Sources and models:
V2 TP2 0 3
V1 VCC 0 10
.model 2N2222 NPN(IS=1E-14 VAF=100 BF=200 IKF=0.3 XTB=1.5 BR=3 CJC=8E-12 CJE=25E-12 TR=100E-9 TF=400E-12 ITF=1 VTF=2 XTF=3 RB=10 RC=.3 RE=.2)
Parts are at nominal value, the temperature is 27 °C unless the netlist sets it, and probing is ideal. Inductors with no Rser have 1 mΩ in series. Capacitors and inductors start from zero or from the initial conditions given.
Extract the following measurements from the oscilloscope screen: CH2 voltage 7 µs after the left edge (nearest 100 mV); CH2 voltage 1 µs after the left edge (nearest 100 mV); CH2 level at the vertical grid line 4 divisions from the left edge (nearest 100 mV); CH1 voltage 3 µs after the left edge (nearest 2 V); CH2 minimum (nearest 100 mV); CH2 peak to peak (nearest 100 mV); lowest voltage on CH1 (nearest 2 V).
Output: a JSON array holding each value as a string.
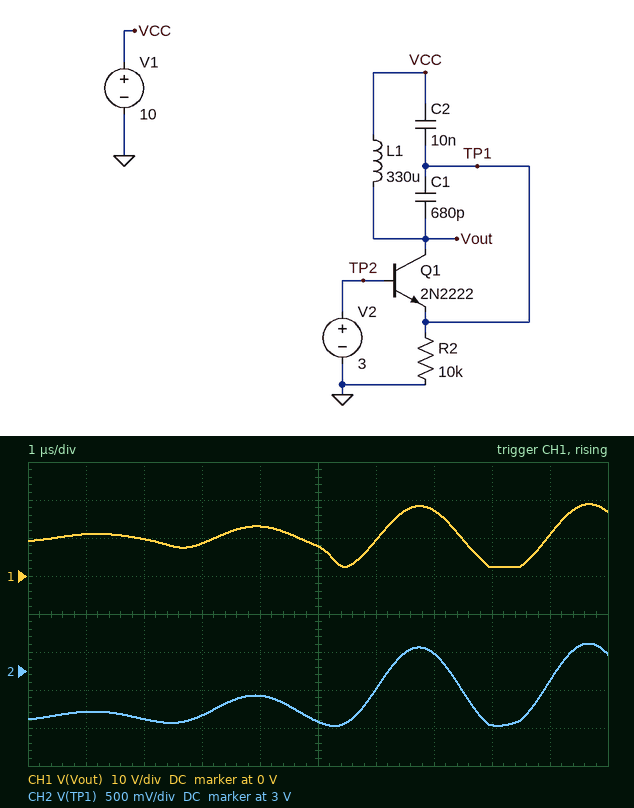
["3.2 V", "2.5 V", "2.7 V", "8 V", "2.3 V", "1.1 V", "2 V"]
